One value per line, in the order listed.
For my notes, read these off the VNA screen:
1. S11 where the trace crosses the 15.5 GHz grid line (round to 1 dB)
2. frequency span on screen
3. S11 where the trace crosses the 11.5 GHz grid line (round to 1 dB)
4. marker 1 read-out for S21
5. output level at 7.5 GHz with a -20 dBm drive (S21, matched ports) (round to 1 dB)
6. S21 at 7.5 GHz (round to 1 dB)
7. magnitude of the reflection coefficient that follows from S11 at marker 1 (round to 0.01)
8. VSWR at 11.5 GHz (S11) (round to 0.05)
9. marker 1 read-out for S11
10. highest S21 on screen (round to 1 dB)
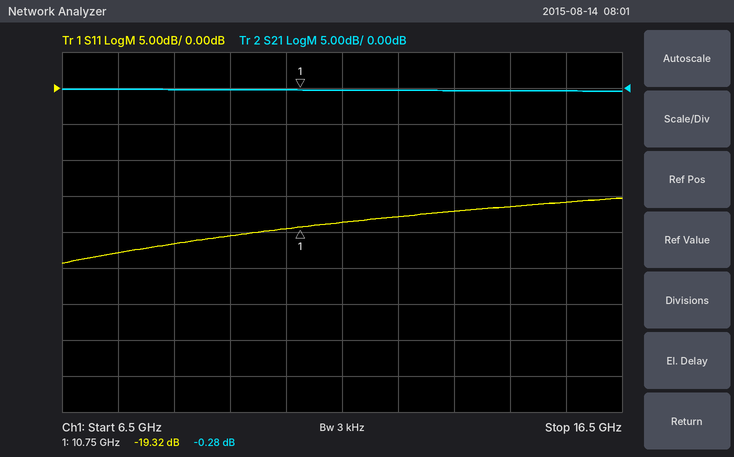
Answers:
-16 dB
10 GHz
-19 dB
-0.28 dB
-20 dBm
0 dB
0.11
1.25
-19.32 dB
0 dB
